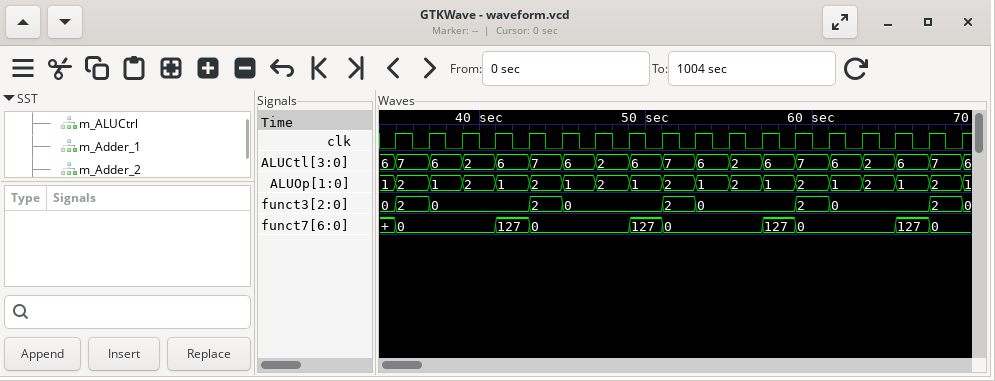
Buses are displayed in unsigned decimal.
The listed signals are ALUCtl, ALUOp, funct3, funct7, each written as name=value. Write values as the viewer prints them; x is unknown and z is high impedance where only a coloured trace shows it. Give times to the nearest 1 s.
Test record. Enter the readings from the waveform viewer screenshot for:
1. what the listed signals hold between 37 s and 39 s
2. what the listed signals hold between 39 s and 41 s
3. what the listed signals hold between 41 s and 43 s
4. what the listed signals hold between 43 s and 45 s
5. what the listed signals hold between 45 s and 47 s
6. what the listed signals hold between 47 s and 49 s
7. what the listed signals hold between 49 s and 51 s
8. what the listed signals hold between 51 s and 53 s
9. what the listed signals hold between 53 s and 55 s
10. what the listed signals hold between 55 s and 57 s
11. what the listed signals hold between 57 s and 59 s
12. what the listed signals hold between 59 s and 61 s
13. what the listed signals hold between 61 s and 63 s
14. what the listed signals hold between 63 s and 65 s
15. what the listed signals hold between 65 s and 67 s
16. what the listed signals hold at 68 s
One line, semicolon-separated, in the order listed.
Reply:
ALUCtl=6, ALUOp=1, funct3=0, funct7=0; ALUCtl=2, ALUOp=2, funct3=0, funct7=0; ALUCtl=6, ALUOp=1, funct3=0, funct7=127; ALUCtl=7, ALUOp=2, funct3=2, funct7=0; ALUCtl=6, ALUOp=1, funct3=0, funct7=0; ALUCtl=2, ALUOp=2, funct3=0, funct7=0; ALUCtl=6, ALUOp=1, funct3=0, funct7=127; ALUCtl=7, ALUOp=2, funct3=2, funct7=0; ALUCtl=6, ALUOp=1, funct3=0, funct7=0; ALUCtl=2, ALUOp=2, funct3=0, funct7=0; ALUCtl=6, ALUOp=1, funct3=0, funct7=127; ALUCtl=7, ALUOp=2, funct3=2, funct7=0; ALUCtl=6, ALUOp=1, funct3=0, funct7=0; ALUCtl=2, ALUOp=2, funct3=0, funct7=0; ALUCtl=6, ALUOp=1, funct3=0, funct7=127; ALUCtl=7, ALUOp=2, funct3=2, funct7=0
